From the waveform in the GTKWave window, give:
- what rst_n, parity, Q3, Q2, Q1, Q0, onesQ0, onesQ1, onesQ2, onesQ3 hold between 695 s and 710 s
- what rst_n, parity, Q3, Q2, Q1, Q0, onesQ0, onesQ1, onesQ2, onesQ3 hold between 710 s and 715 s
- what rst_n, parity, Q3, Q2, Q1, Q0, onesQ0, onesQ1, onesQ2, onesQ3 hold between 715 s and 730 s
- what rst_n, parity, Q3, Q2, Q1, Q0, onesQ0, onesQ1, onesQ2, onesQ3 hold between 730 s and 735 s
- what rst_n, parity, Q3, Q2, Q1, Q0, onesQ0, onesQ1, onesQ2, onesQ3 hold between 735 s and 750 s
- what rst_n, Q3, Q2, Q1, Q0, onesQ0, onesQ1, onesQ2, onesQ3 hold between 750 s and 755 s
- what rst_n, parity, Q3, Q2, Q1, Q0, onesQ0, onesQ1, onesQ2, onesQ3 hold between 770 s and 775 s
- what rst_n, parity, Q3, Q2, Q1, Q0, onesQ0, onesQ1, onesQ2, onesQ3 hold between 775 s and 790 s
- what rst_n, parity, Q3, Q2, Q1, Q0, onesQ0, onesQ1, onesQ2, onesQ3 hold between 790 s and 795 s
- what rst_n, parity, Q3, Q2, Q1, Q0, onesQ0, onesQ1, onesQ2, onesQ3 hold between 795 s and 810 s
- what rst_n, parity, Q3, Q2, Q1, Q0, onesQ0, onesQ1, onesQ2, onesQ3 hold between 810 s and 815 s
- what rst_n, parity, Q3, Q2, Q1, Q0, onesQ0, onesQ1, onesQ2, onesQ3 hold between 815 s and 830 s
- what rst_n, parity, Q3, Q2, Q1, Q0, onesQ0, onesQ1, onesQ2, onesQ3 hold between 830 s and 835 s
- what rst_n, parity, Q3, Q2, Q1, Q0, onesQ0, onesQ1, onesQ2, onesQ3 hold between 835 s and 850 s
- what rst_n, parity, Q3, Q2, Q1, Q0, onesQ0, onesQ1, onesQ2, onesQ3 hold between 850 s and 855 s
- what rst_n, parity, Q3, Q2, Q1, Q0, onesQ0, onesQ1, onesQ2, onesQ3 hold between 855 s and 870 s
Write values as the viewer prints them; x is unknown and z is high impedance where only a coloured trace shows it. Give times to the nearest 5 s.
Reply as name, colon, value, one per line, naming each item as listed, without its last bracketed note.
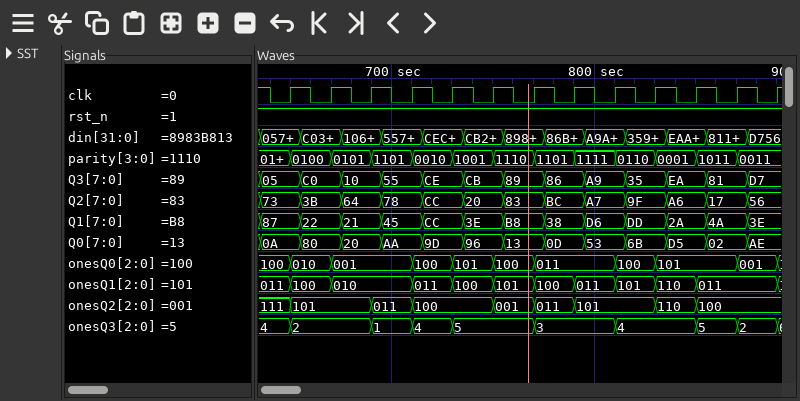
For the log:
what rst_n, parity, Q3, Q2, Q1, Q0, onesQ0, onesQ1, onesQ2, onesQ3 hold between 695 s and 710 s: rst_n=1, parity=1101, Q3=55, Q2=78, Q1=45, Q0=AA, onesQ0=001, onesQ1=010, onesQ2=011, onesQ3=1
what rst_n, parity, Q3, Q2, Q1, Q0, onesQ0, onesQ1, onesQ2, onesQ3 hold between 710 s and 715 s: rst_n=1, parity=0010, Q3=55, Q2=78, Q1=45, Q0=AA, onesQ0=100, onesQ1=011, onesQ2=100, onesQ3=4
what rst_n, parity, Q3, Q2, Q1, Q0, onesQ0, onesQ1, onesQ2, onesQ3 hold between 715 s and 730 s: rst_n=1, parity=0010, Q3=CE, Q2=CC, Q1=CC, Q0=9D, onesQ0=100, onesQ1=011, onesQ2=100, onesQ3=4
what rst_n, parity, Q3, Q2, Q1, Q0, onesQ0, onesQ1, onesQ2, onesQ3 hold between 730 s and 735 s: rst_n=1, parity=1001, Q3=CE, Q2=CC, Q1=CC, Q0=9D, onesQ0=101, onesQ1=100, onesQ2=100, onesQ3=5
what rst_n, parity, Q3, Q2, Q1, Q0, onesQ0, onesQ1, onesQ2, onesQ3 hold between 735 s and 750 s: rst_n=1, parity=1001, Q3=CB, Q2=20, Q1=3E, Q0=96, onesQ0=101, onesQ1=100, onesQ2=100, onesQ3=5
what rst_n, Q3, Q2, Q1, Q0, onesQ0, onesQ1, onesQ2, onesQ3 hold between 750 s and 755 s: rst_n=1, Q3=CB, Q2=20, Q1=3E, Q0=96, onesQ0=100, onesQ1=101, onesQ2=001, onesQ3=5
what rst_n, parity, Q3, Q2, Q1, Q0, onesQ0, onesQ1, onesQ2, onesQ3 hold between 770 s and 775 s: rst_n=1, parity=1101, Q3=89, Q2=83, Q1=B8, Q0=13, onesQ0=011, onesQ1=100, onesQ2=011, onesQ3=3
what rst_n, parity, Q3, Q2, Q1, Q0, onesQ0, onesQ1, onesQ2, onesQ3 hold between 775 s and 790 s: rst_n=1, parity=1101, Q3=86, Q2=BC, Q1=38, Q0=0D, onesQ0=011, onesQ1=100, onesQ2=011, onesQ3=3
what rst_n, parity, Q3, Q2, Q1, Q0, onesQ0, onesQ1, onesQ2, onesQ3 hold between 790 s and 795 s: rst_n=1, parity=1111, Q3=86, Q2=BC, Q1=38, Q0=0D, onesQ0=011, onesQ1=011, onesQ2=101, onesQ3=3
what rst_n, parity, Q3, Q2, Q1, Q0, onesQ0, onesQ1, onesQ2, onesQ3 hold between 795 s and 810 s: rst_n=1, parity=1111, Q3=A9, Q2=A7, Q1=D6, Q0=53, onesQ0=011, onesQ1=011, onesQ2=101, onesQ3=3
what rst_n, parity, Q3, Q2, Q1, Q0, onesQ0, onesQ1, onesQ2, onesQ3 hold between 810 s and 815 s: rst_n=1, parity=0110, Q3=A9, Q2=A7, Q1=D6, Q0=53, onesQ0=100, onesQ1=101, onesQ2=101, onesQ3=4
what rst_n, parity, Q3, Q2, Q1, Q0, onesQ0, onesQ1, onesQ2, onesQ3 hold between 815 s and 830 s: rst_n=1, parity=0110, Q3=35, Q2=9F, Q1=DD, Q0=6B, onesQ0=100, onesQ1=101, onesQ2=101, onesQ3=4
what rst_n, parity, Q3, Q2, Q1, Q0, onesQ0, onesQ1, onesQ2, onesQ3 hold between 830 s and 835 s: rst_n=1, parity=0001, Q3=35, Q2=9F, Q1=DD, Q0=6B, onesQ0=101, onesQ1=110, onesQ2=110, onesQ3=4
what rst_n, parity, Q3, Q2, Q1, Q0, onesQ0, onesQ1, onesQ2, onesQ3 hold between 835 s and 850 s: rst_n=1, parity=0001, Q3=EA, Q2=A6, Q1=2A, Q0=D5, onesQ0=101, onesQ1=110, onesQ2=110, onesQ3=4
what rst_n, parity, Q3, Q2, Q1, Q0, onesQ0, onesQ1, onesQ2, onesQ3 hold between 850 s and 855 s: rst_n=1, parity=1011, Q3=EA, Q2=A6, Q1=2A, Q0=D5, onesQ0=101, onesQ1=011, onesQ2=100, onesQ3=5
what rst_n, parity, Q3, Q2, Q1, Q0, onesQ0, onesQ1, onesQ2, onesQ3 hold between 855 s and 870 s: rst_n=1, parity=1011, Q3=81, Q2=17, Q1=4A, Q0=02, onesQ0=101, onesQ1=011, onesQ2=100, onesQ3=5
